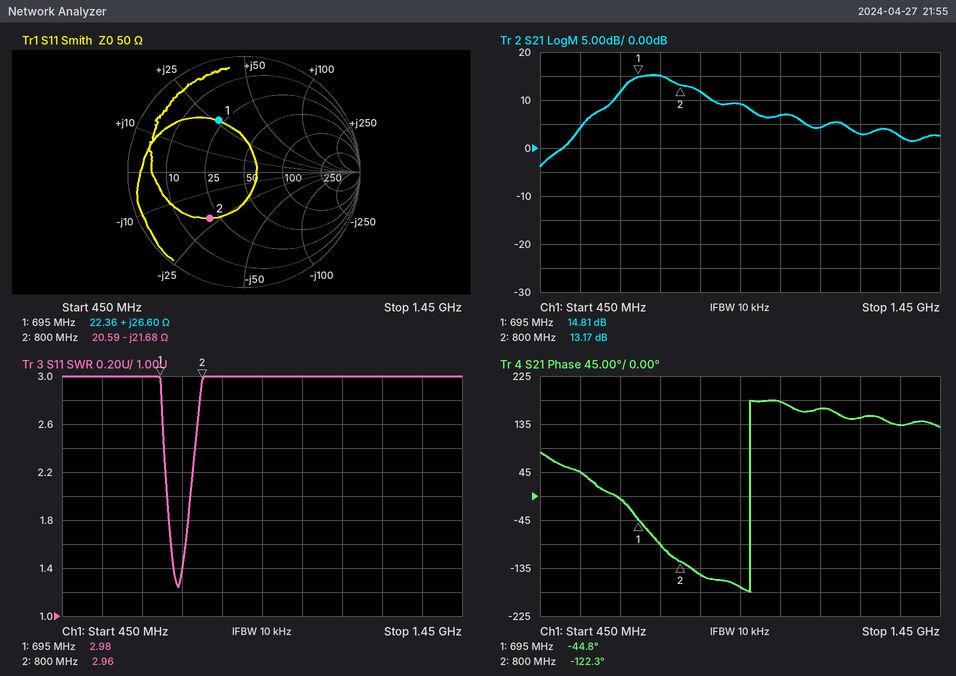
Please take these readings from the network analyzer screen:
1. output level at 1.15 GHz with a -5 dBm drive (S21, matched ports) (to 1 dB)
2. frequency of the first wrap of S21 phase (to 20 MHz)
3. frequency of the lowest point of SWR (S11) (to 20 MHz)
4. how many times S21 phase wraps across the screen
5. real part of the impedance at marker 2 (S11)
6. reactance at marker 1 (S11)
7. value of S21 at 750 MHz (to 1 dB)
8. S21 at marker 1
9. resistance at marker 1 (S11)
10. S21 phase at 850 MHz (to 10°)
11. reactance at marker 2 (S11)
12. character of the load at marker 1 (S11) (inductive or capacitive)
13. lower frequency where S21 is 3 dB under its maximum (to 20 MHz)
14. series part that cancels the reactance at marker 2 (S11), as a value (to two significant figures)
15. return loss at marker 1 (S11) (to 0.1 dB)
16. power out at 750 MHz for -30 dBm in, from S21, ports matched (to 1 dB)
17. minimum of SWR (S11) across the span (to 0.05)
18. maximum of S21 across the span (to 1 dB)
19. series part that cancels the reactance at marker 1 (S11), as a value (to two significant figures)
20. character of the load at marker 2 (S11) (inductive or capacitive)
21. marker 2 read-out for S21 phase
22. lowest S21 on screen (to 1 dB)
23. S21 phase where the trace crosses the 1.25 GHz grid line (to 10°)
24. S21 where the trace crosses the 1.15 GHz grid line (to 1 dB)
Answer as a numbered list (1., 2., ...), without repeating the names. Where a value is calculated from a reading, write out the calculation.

1. -5 dBm + (4 dB) = -1 dBm
2. 980 MHz
3. 740 MHz
4. 1
5. 20.59 Ω
6. +26.60 Ω
7. 15 dB
8. 14.81 dB
9. 22.36 Ω
10. -150°
11. -21.68 Ω
12. inductive
13. 660 MHz
14. L = 21.68 Ω/(2π × 800 MHz) ≈ 4.3 nH
15. 6.1 dB
16. -30 dBm + (15 dB) = -15 dBm
17. 1.25
18. 15 dB
19. C = 1/(2π × 695 MHz × 26.6 Ω) ≈ 8.6 pF
20. capacitive
21. -122.3°
22. -4 dB
23. 150°
24. 4 dB
